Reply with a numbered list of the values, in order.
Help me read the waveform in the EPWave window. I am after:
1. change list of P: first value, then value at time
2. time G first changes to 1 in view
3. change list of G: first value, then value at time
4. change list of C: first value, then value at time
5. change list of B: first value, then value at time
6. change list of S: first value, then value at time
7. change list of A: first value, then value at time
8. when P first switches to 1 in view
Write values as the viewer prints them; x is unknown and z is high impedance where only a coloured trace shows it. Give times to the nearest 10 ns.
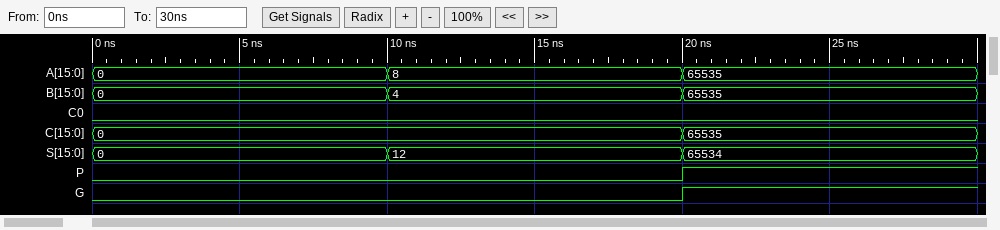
1. 0, 1 at 20 ns
2. 20 ns
3. 0, 1 at 20 ns
4. 0, 65535 at 20 ns
5. 0, 4 at 10 ns, 65535 at 20 ns
6. 0, 12 at 10 ns, 65534 at 20 ns
7. 0, 8 at 10 ns, 65535 at 20 ns
8. 20 ns
